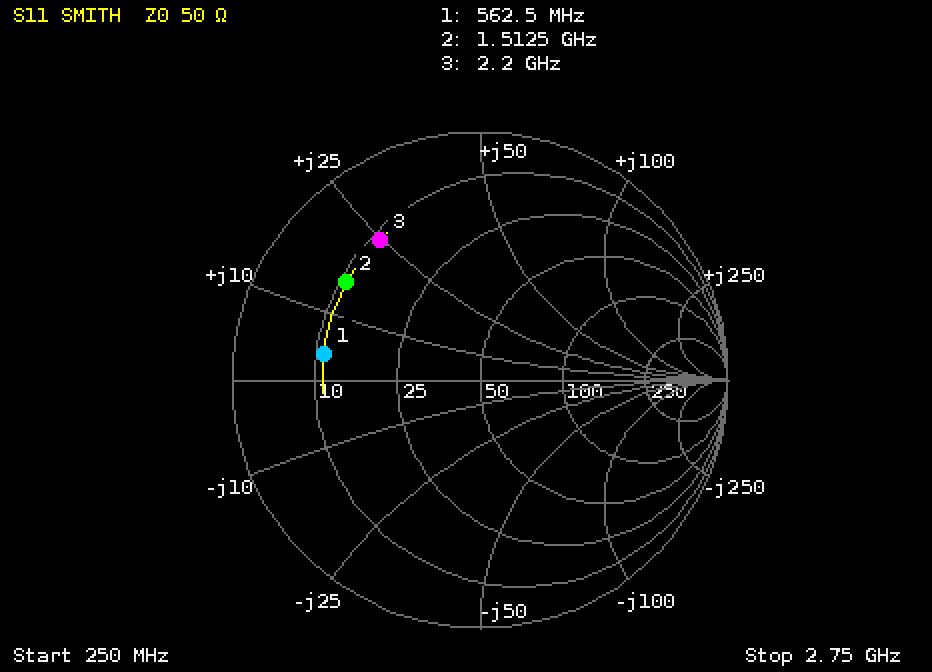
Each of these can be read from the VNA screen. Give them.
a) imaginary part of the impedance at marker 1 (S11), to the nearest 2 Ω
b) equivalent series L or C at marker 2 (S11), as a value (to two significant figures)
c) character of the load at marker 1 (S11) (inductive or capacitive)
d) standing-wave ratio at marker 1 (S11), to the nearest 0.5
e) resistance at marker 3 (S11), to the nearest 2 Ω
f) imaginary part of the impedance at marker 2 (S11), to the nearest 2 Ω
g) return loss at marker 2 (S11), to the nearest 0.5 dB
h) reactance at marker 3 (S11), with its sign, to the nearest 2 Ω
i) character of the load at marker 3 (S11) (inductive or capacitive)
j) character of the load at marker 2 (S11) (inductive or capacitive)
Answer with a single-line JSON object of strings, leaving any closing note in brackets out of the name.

{"imaginary part of the impedance at marker 1 (S11), to the nearest 2 Ω": "+4 Ω", "equivalent series L or C at marker 2 (S11), as a value": "1.7 nH", "character of the load at marker 1 (S11)": "inductive", "standing-wave ratio at marker 1 (S11), to the nearest 0.5": "4.5", "resistance at marker 3 (S11), to the nearest 2 Ω": "12 Ω", "imaginary part of the impedance at marker 2 (S11), to the nearest 2 Ω": "+16 Ω", "return loss at marker 2 (S11), to the nearest 0.5 dB": "3.5 dB", "reactance at marker 3 (S11), with its sign, to the nearest 2 Ω": "+24 Ω", "character of the load at marker 3 (S11)": "inductive", "character of the load at marker 2 (S11)": "inductive"}
